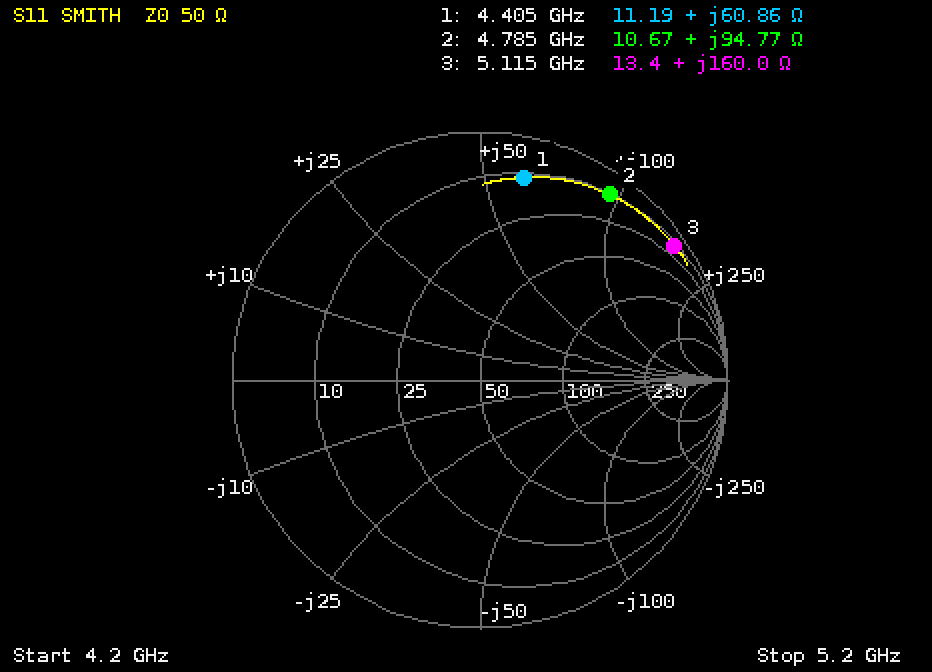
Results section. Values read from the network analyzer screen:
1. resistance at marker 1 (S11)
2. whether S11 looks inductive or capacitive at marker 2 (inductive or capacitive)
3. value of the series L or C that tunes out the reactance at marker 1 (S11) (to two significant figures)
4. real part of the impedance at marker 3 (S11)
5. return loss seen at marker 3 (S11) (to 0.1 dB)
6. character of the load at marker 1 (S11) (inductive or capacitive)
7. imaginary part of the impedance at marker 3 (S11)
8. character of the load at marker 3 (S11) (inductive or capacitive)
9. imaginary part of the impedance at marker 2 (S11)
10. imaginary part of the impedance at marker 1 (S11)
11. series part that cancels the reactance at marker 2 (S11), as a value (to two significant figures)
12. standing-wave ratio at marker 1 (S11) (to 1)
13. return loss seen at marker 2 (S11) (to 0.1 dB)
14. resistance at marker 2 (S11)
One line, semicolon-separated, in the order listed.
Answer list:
11.19 Ω; inductive; 590 fF; 13.4 Ω; 0.4 dB; inductive; +160.0 Ω; inductive; +94.77 Ω; +60.86 Ω; 350 fF; 11; 0.8 dB; 10.67 Ω
